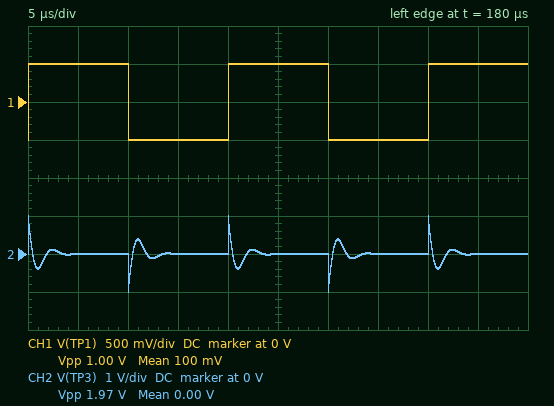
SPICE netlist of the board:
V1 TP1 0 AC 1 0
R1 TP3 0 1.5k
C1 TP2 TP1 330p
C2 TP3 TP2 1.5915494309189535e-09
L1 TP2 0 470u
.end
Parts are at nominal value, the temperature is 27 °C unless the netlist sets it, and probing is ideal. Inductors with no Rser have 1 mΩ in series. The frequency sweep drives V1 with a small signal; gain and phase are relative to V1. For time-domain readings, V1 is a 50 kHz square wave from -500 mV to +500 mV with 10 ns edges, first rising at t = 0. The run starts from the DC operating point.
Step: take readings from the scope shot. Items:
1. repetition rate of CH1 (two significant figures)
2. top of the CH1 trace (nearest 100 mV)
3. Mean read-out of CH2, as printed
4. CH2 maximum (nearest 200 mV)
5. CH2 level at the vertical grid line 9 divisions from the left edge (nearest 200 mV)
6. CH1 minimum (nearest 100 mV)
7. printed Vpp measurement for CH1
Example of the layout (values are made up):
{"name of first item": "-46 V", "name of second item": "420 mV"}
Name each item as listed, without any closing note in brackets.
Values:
{"repetition rate of CH1": "50 kHz", "top of the CH1 trace": "500 mV", "Mean read-out of CH2, as printed": "0.00 V", "CH2 maximum": "1.0 V", "CH2 level at the vertical grid line 9 divisions from the left edge": "0 V", "CH1 minimum": "-500 mV", "printed Vpp measurement for CH1": "1.00 V"}
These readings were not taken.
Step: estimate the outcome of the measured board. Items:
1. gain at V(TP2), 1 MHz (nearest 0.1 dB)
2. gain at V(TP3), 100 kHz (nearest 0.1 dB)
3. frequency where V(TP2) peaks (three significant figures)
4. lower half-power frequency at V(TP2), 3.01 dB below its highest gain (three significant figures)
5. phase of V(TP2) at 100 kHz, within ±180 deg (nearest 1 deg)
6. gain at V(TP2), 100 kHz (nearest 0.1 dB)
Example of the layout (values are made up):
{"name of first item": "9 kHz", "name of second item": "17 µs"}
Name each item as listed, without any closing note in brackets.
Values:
{"gain at V(TP2), 1 MHz": "0.8 dB", "gain at V(TP3), 100 kHz": "-24.5 dB", "frequency where V(TP2) peaks": "462 kHz", "lower half-power frequency at V(TP2), 3.01 dB below its highest gain": "315 kHz", "phase of V(TP2) at 100 kHz, within ±180 deg": "171 deg", "gain at V(TP2), 100 kHz": "-22.9 dB"}
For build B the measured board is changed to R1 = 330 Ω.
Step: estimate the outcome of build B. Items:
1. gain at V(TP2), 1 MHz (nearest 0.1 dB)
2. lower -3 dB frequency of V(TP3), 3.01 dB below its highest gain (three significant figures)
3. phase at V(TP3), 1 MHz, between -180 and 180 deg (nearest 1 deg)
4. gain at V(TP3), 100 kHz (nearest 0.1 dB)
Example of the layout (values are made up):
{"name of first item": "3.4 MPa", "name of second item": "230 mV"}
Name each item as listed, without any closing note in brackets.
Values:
{"gain at V(TP2), 1 MHz": "-5.2 dB", "lower -3 dB frequency of V(TP3), 3.01 dB below its highest gain": "1.65 MHz", "phase at V(TP3), 1 MHz, between -180 and 180 deg": "64 deg", "gain at V(TP3), 100 kHz": "-31.0 dB"}
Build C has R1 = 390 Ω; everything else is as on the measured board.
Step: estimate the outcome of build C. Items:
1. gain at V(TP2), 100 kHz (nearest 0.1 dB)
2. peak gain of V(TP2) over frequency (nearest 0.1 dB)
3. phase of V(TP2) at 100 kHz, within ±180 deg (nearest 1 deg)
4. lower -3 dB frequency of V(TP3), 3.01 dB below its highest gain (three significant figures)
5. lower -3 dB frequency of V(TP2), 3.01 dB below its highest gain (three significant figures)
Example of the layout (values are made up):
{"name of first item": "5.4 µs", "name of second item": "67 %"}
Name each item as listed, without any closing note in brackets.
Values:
{"gain at V(TP2), 100 kHz": "-21.0 dB", "peak gain of V(TP2) over frequency": "0 dB", "phase of V(TP2) at 100 kHz, within ±180 deg": "172 deg", "lower -3 dB frequency of V(TP3), 3.01 dB below its highest gain": "1.36 MHz", "lower -3 dB frequency of V(TP2), 3.01 dB below its highest gain": "1.31 MHz"}
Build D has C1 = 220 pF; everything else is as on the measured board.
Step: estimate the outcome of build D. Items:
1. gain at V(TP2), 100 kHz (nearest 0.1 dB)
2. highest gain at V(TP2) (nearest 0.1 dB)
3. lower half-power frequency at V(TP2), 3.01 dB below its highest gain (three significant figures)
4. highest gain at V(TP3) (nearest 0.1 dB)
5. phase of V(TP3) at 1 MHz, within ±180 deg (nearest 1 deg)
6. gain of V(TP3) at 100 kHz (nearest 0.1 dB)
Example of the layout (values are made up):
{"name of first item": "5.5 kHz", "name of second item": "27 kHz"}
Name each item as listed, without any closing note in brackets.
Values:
{"gain at V(TP2), 100 kHz": "-26.7 dB", "highest gain at V(TP2)": "1.1 dB", "lower half-power frequency at V(TP2), 3.01 dB below its highest gain": "393 kHz", "highest gain at V(TP3)": "1.0 dB", "phase of V(TP3) at 1 MHz, within ±180 deg": "35 deg", "gain of V(TP3) at 100 kHz": "-28.3 dB"}
